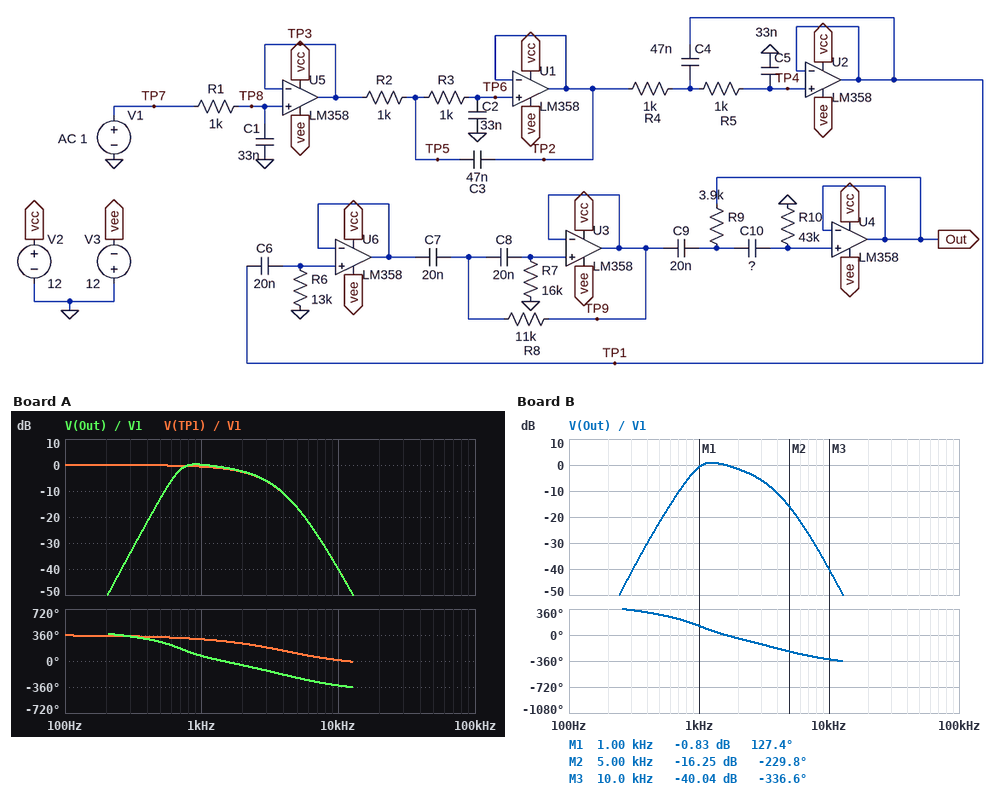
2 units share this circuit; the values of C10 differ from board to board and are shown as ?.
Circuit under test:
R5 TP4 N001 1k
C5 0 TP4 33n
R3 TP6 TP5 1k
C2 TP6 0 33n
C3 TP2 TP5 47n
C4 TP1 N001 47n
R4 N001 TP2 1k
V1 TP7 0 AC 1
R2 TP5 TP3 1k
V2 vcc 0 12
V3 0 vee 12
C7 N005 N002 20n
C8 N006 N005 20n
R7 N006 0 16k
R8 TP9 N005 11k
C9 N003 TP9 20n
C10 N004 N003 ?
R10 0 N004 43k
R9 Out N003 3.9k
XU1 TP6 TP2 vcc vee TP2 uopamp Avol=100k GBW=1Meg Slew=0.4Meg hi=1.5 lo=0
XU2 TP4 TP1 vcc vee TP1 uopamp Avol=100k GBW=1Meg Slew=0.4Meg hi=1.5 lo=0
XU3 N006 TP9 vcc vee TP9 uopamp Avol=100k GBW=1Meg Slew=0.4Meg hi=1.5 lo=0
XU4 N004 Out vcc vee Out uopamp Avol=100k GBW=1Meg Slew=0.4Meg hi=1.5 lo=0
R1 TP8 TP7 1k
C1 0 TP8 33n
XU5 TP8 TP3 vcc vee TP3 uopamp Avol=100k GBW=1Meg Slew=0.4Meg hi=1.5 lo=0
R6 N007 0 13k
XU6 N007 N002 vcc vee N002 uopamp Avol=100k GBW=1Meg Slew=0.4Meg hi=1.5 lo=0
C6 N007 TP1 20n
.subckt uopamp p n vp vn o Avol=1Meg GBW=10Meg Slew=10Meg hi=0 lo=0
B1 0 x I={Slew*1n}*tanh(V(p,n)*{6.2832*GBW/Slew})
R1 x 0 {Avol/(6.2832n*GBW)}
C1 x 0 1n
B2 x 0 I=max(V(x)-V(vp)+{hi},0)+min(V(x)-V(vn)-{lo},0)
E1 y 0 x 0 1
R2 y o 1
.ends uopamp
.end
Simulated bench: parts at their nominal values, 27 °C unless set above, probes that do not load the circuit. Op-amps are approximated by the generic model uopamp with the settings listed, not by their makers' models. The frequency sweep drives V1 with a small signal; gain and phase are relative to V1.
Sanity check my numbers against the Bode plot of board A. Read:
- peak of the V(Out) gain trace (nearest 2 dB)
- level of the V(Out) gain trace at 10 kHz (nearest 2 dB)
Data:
0 dB
-40 dB
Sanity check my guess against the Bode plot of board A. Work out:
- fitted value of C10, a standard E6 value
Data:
15 nF
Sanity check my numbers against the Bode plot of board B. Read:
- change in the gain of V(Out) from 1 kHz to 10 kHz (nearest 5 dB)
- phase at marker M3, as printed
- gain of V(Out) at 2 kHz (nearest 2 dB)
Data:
-40 dB
-336.6 deg
-2 dB
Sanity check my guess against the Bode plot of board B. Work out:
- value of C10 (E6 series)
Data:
6.8 nF
